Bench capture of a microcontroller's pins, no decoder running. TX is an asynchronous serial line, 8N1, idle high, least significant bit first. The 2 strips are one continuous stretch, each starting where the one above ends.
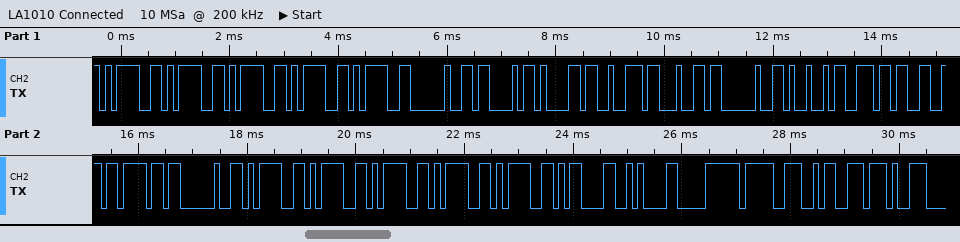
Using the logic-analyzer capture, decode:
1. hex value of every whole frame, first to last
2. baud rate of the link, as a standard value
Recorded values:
3D 3D 3D 3D 3D 20 43 61 72 64 20 49 6E 66 6F 20 3D 3D 3D 3D 3D 0D 0A F0 9F 9A 97
9600 baud
